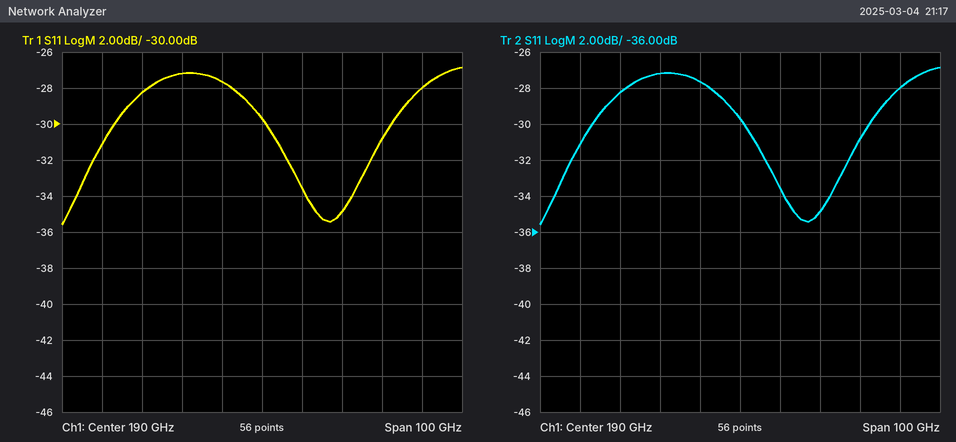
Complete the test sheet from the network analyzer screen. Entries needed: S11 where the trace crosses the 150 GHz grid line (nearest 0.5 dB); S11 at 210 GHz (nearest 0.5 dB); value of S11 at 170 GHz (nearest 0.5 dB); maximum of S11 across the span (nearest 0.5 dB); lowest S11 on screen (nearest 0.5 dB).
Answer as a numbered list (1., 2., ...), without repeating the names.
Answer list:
1. -31.0 dB
2. -35.0 dB
3. -27.0 dB
4. -27.0 dB
5. -35.5 dB
